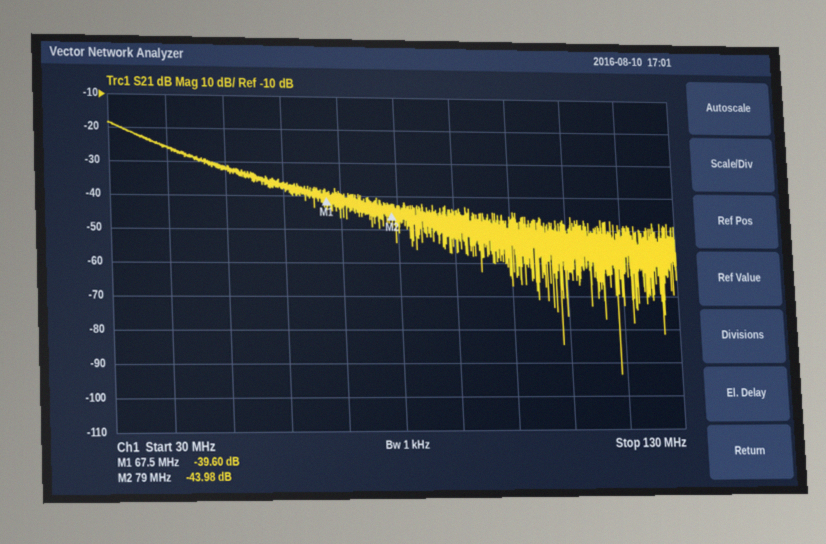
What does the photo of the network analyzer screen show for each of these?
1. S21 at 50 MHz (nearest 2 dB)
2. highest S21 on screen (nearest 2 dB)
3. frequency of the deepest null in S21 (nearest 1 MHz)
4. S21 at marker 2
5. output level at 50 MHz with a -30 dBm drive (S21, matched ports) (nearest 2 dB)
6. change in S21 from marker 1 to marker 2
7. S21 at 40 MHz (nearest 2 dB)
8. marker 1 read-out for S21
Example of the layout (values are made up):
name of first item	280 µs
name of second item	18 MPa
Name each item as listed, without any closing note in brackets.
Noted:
S21 at 50 MHz	-32 dB
highest S21 on screen	-18 dB
frequency of the deepest null in S21	119 MHz
S21 at marker 2	-43.98 dB
output level at 50 MHz with a -30 dBm drive (S21, matched ports)	-62 dBm
change in S21 from marker 1 to marker 2	-4.38 dB
S21 at 40 MHz	-26 dB
marker 1 read-out for S21	-39.60 dB
